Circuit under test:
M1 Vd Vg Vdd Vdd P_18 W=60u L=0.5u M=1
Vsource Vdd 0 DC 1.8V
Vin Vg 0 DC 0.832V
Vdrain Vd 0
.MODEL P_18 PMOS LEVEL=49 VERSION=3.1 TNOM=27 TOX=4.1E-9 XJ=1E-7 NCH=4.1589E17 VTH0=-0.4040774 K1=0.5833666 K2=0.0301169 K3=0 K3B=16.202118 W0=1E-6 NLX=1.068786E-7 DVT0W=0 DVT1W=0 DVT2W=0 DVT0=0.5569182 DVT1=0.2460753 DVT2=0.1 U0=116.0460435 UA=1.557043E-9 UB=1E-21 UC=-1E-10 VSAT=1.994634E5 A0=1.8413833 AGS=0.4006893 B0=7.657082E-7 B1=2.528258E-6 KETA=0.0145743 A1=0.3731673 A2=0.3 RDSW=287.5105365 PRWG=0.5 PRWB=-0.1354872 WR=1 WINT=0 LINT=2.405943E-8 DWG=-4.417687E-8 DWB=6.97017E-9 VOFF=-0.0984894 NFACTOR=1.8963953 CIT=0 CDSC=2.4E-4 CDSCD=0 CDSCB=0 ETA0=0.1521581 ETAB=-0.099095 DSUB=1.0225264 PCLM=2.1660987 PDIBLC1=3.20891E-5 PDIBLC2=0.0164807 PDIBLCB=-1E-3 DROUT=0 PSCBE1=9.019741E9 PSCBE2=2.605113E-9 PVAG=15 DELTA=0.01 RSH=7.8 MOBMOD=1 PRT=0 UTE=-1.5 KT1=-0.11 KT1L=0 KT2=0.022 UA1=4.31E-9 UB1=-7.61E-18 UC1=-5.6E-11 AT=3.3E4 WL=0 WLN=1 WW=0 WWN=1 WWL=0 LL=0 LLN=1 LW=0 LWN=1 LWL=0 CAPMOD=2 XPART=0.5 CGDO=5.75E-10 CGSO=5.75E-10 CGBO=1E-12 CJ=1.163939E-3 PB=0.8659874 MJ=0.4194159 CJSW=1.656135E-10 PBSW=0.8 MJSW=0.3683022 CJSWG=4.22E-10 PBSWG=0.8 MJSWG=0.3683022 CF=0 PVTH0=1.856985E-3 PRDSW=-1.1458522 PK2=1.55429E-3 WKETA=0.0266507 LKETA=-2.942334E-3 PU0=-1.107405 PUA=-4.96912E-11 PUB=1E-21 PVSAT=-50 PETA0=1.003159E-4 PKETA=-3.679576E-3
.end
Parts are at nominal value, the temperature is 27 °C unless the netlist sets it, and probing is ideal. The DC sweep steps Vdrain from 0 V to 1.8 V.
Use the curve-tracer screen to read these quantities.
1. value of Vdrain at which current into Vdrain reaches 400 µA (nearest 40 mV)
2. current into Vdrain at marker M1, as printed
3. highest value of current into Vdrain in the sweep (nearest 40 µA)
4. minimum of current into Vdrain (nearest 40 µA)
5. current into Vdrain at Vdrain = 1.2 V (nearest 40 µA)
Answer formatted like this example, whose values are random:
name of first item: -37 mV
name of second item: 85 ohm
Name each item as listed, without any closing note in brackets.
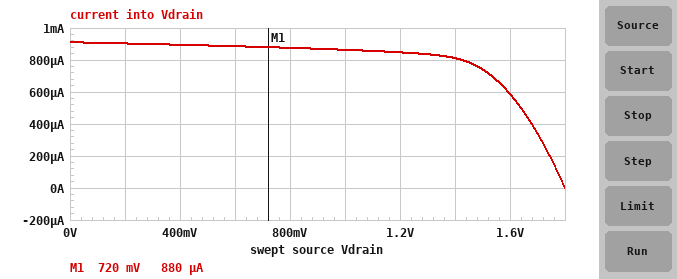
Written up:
value of Vdrain at which current into Vdrain reaches 400 µA: 1.68 V
current into Vdrain at marker M1, as printed: 880 µA
highest value of current into Vdrain in the sweep: 920 µA
minimum of current into Vdrain: 0 A
current into Vdrain at Vdrain = 1.2 V: 840 µA
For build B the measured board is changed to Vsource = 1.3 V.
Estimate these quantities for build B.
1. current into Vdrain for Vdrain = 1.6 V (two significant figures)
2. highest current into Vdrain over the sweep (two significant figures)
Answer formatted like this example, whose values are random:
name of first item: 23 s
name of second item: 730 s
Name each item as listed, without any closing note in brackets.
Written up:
current into Vdrain for Vdrain = 1.6 V: -520 µA
highest current into Vdrain over the sweep: 12 µA
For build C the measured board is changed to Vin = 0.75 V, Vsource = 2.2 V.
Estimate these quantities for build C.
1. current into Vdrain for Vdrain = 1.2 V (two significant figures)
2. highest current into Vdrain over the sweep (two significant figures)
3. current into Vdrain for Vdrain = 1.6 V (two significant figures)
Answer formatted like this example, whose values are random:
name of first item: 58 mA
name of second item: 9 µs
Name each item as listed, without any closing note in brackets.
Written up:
current into Vdrain for Vdrain = 1.2 V: 2.7 mA
highest current into Vdrain over the sweep: 2.8 mA
current into Vdrain for Vdrain = 1.6 V: 2.4 mA
